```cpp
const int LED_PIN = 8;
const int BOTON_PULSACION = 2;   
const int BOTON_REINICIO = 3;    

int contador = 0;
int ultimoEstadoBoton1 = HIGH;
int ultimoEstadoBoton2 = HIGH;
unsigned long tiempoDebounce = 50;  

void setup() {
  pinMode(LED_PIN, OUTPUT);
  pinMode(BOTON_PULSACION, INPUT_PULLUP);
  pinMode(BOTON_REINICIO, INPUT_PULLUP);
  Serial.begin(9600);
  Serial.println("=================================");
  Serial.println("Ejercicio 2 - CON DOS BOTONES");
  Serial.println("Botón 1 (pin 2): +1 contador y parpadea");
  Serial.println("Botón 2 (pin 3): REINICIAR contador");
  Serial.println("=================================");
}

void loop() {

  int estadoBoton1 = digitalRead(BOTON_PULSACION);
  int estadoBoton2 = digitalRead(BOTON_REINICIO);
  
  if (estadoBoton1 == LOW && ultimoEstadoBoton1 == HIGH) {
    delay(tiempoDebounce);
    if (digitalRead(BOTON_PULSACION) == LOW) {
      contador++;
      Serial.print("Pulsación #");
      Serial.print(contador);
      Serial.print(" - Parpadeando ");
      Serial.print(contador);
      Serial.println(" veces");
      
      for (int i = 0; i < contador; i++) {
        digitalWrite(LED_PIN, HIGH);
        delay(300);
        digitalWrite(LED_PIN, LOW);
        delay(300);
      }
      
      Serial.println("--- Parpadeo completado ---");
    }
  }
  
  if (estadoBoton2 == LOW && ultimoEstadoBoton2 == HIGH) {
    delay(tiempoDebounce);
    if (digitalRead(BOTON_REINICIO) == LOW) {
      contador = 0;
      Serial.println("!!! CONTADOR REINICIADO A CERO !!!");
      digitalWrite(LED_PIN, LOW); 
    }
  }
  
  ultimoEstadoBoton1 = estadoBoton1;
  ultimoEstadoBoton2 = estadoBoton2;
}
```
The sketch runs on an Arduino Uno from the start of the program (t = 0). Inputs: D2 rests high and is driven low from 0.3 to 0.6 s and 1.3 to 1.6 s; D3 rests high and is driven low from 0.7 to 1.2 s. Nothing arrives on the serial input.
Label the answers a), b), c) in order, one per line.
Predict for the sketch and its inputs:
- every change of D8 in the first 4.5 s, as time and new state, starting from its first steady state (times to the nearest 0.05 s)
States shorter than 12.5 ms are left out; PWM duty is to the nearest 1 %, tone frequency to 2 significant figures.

a) 0 s low; 0.35 s high; 0.65 s low; 1.35 s high; 1.65 s low
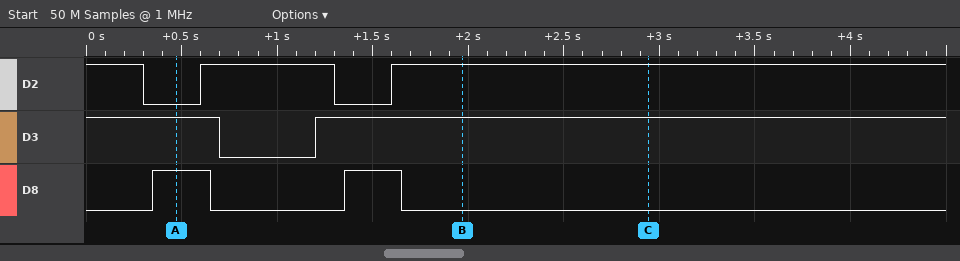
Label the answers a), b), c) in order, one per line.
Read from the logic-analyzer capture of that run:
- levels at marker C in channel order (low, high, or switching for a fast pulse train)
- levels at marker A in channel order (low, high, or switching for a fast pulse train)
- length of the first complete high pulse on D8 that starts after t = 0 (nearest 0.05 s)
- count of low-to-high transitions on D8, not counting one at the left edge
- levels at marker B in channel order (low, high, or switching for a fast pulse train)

a) D2 high, D3 high, D8 low
b) D2 low, D3 high, D8 high
c) 0.30 s
d) 2
e) D2 high, D3 high, D8 low
